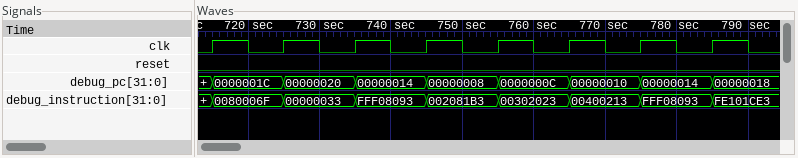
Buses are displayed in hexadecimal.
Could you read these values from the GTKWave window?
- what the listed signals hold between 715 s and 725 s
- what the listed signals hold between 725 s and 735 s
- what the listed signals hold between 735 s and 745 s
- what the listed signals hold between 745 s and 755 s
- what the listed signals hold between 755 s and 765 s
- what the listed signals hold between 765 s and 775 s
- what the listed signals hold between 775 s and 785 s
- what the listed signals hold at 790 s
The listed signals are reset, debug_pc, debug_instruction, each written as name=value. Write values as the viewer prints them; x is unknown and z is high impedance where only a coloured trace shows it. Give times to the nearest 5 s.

reset=0, debug_pc=0000001C, debug_instruction=0080006F
reset=0, debug_pc=00000020, debug_instruction=00000033
reset=0, debug_pc=00000014, debug_instruction=FFF08093
reset=0, debug_pc=00000008, debug_instruction=002081B3
reset=0, debug_pc=0000000C, debug_instruction=00302023
reset=0, debug_pc=00000010, debug_instruction=00400213
reset=0, debug_pc=00000014, debug_instruction=FFF08093
reset=0, debug_pc=00000018, debug_instruction=FE101CE3
